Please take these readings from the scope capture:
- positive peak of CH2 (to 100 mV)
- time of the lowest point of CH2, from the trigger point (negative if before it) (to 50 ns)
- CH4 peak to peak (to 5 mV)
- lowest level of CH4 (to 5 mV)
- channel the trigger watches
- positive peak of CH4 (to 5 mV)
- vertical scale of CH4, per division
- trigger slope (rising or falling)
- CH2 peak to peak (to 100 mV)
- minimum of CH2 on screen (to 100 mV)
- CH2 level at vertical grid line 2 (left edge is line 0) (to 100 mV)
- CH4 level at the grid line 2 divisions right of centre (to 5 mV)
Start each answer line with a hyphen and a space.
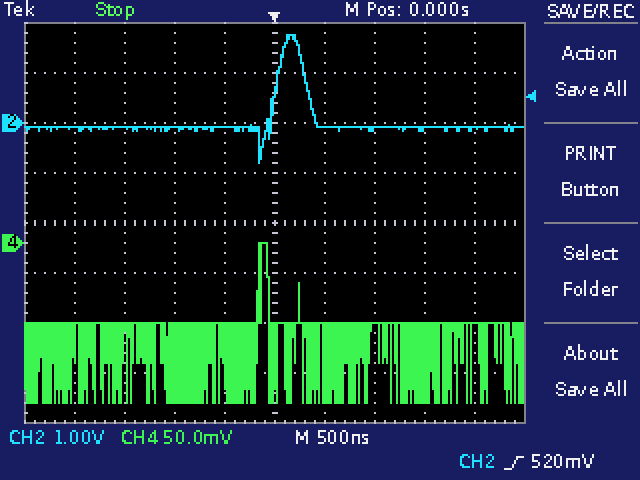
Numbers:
- 1.8 V
- -150 ns
- 160 mV
- -160 mV
- CH2
- 0 mV
- 50 mV
- rising
- 2.6 V
- -800 mV
- -100 mV
- -85 mV
